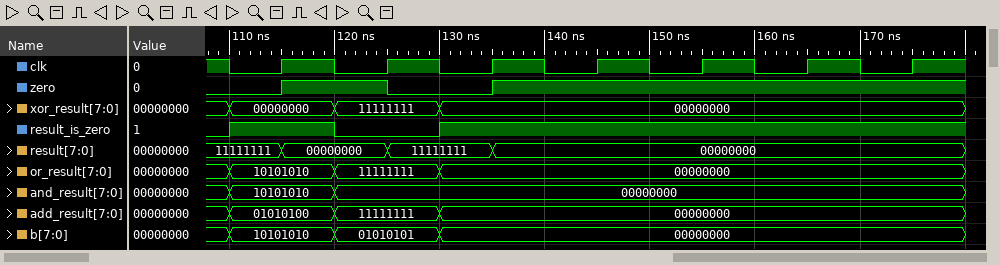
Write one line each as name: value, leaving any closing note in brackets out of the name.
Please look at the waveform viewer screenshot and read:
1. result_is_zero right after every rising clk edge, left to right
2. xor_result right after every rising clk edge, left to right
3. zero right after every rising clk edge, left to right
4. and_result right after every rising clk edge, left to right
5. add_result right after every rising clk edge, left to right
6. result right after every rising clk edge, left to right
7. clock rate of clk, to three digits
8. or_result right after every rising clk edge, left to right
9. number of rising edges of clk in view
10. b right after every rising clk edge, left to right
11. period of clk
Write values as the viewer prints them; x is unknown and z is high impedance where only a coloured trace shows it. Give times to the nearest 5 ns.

result_is_zero right after every rising clk edge, left to right: 1 0 1 1 1 1 1
xor_result right after every rising clk edge, left to right: 00000000, 11111111, 00000000, 00000000, 00000000, 00000000, 00000000
zero right after every rising clk edge, left to right: 1 0 1 1 1 1 1
and_result right after every rising clk edge, left to right: 10101010, 00000000, 00000000, 00000000, 00000000, 00000000, 00000000
add_result right after every rising clk edge, left to right: 01010100, 11111111, 00000000, 00000000, 00000000, 00000000, 00000000
result right after every rising clk edge, left to right: 00000000, 11111111, 00000000, 00000000, 00000000, 00000000, 00000000
clock rate of clk, to three digits: 100 MHz
or_result right after every rising clk edge, left to right: 10101010, 11111111, 00000000, 00000000, 00000000, 00000000, 00000000
number of rising edges of clk in view: 7
b right after every rising clk edge, left to right: 10101010, 01010101, 00000000, 00000000, 00000000, 00000000, 00000000
period of clk: 10 ns
